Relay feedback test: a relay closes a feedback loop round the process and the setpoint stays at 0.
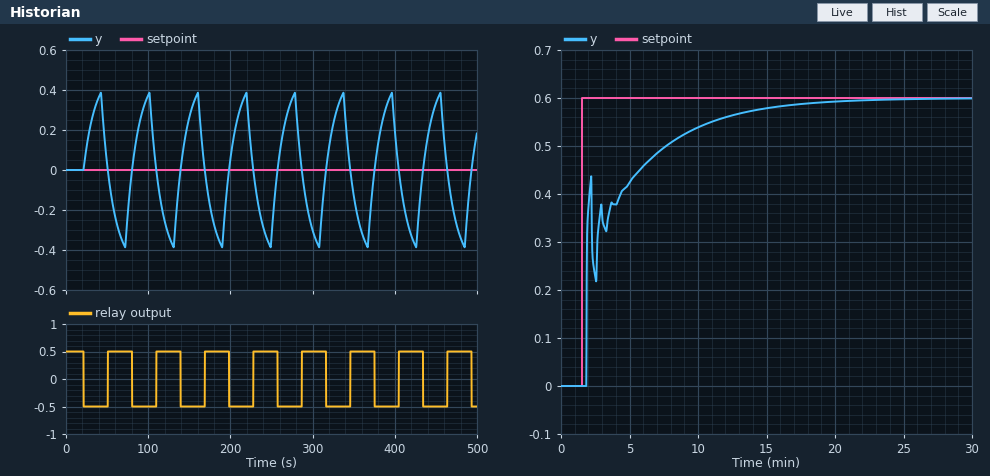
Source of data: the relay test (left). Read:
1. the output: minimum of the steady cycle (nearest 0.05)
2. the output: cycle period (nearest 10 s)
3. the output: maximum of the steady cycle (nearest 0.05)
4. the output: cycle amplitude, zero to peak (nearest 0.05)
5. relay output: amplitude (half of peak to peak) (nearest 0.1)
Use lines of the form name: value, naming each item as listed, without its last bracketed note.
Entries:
the output: minimum of the steady cycle: -0.40
the output: cycle period: 60 s
the output: maximum of the steady cycle: 0.40
the output: cycle amplitude, zero to peak: 0.40
relay output: amplitude (half of peak to peak): 0.5
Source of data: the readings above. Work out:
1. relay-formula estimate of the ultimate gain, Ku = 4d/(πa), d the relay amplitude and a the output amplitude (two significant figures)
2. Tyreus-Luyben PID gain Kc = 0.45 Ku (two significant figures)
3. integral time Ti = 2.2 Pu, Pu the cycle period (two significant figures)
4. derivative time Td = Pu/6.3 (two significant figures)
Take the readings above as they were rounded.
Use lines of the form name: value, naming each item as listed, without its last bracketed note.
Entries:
relay-formula estimate of the ultimate gain, Ku = 4d/(πa), d the relay amplitude and a the output amplitude: 1.6
Tyreus-Luyben PID gain Kc = 0.45 Ku: 0.72
integral time Ti = 2.2 Pu, Pu the cycle period: 130 s
derivative time Td = Pu/6.3: 9.5 s
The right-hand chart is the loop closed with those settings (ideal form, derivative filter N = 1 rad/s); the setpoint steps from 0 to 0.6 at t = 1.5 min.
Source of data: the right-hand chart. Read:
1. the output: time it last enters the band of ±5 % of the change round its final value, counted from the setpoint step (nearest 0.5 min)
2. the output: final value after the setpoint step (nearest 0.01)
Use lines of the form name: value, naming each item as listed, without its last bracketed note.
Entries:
the output: time it last enters the band of ±5 % of the change round its final value, counted from the setpoint step: 12.0 min
the output: final value after the setpoint step: 0.60
